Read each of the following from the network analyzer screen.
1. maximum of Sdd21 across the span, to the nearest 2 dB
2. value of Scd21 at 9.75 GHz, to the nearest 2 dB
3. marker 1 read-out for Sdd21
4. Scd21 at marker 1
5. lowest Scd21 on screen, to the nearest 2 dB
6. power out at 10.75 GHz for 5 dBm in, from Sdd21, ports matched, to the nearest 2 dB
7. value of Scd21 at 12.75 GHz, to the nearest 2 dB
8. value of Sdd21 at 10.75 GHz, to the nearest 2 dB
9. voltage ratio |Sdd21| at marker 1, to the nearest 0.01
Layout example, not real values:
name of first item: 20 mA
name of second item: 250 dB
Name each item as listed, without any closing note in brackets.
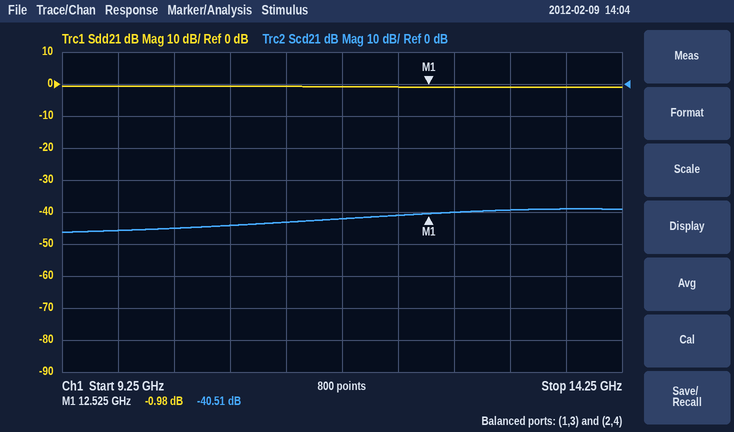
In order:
maximum of Sdd21 across the span, to the nearest 2 dB: 0 dB
value of Scd21 at 9.75 GHz, to the nearest 2 dB: -46 dB
marker 1 read-out for Sdd21: -0.98 dB
Scd21 at marker 1: -40.51 dB
lowest Scd21 on screen, to the nearest 2 dB: -46 dB
power out at 10.75 GHz for 5 dBm in, from Sdd21, ports matched, to the nearest 2 dB: 4 dBm
value of Scd21 at 12.75 GHz, to the nearest 2 dB: -40 dB
value of Sdd21 at 10.75 GHz, to the nearest 2 dB: 0 dB
voltage ratio |Sdd21| at marker 1, to the nearest 0.01: 0.89
